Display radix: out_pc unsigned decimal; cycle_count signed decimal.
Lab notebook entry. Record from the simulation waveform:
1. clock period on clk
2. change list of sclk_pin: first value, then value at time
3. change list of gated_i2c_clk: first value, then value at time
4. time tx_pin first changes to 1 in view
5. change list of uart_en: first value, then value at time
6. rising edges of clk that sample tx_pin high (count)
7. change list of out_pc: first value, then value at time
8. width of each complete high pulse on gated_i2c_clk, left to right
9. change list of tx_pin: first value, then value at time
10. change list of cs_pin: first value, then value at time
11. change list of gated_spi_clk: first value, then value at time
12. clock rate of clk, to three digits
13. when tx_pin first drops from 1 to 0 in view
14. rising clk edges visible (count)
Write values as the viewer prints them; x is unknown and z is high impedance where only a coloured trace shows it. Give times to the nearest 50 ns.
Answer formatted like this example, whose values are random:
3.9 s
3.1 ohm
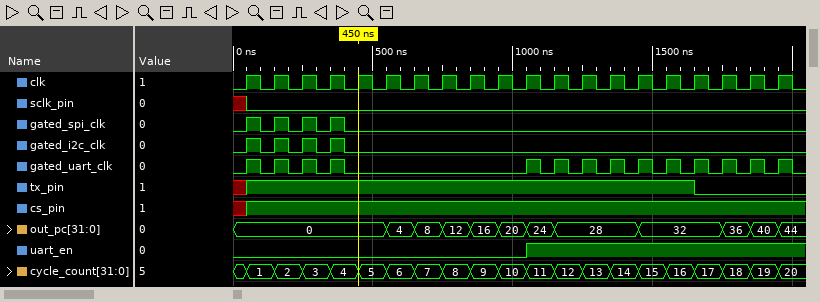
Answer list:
100 ns
x, 0 at 50 ns
0, 1 at 50 ns, 0 at 100 ns, 1 at 150 ns, 0 at 200 ns, 1 at 250 ns, 0 at 300 ns, 1 at 350 ns, 0 at 400 ns
50 ns
0, 1 at 1050 ns
16
0, 4 at 550 ns, 8 at 650 ns, 12 at 750 ns, 16 at 850 ns, 20 at 950 ns, 24 at 1050 ns, 28 at 1150 ns, 32 at 1450 ns, 36 at 1750 ns, 40 at 1850 ns, 44 at 1950 ns
50 ns, 50 ns, 50 ns, 50 ns
x, 1 at 50 ns, 0 at 1650 ns
x, 1 at 50 ns
0, 1 at 50 ns, 0 at 100 ns, 1 at 150 ns, 0 at 200 ns, 1 at 250 ns, 0 at 300 ns, 1 at 350 ns, 0 at 400 ns
10.0 MHz
1650 ns
20
